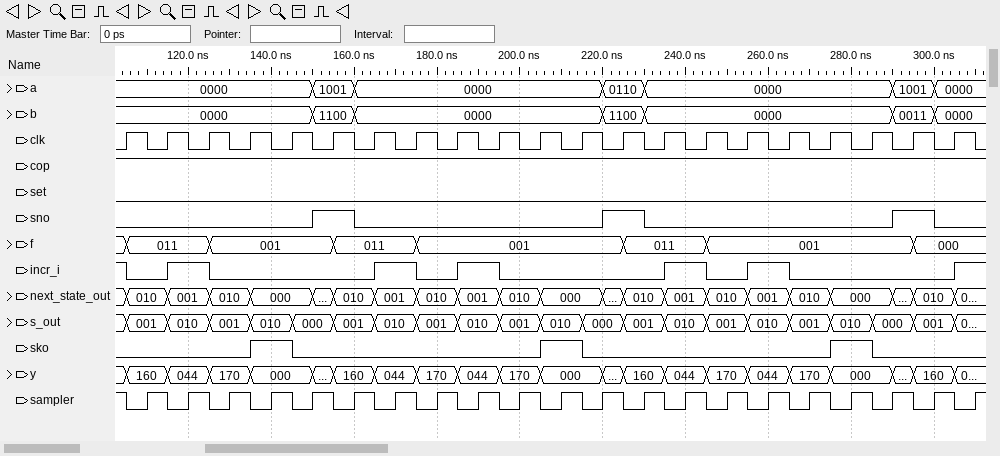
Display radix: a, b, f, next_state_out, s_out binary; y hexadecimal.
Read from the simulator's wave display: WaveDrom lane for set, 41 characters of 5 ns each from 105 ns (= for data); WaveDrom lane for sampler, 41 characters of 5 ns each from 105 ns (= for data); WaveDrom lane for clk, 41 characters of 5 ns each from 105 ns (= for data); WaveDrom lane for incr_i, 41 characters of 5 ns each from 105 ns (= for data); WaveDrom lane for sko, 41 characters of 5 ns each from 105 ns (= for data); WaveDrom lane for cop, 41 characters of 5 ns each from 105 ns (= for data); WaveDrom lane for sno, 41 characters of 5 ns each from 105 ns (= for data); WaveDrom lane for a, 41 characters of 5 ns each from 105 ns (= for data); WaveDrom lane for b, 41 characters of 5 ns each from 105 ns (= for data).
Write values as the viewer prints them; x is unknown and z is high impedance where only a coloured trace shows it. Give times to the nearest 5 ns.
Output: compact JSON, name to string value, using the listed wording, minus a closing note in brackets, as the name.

{"WaveDrom lane for set, 41 characters of 5 ns each from 105 ns": "{name: 'set', wave: '0........................................'}", "WaveDrom lane for sampler, 41 characters of 5 ns each from 105 ns": "{name: 'sampler', wave: '01010101010101010101010101010101010101010'}", "WaveDrom lane for clk, 41 characters of 5 ns each from 105 ns": "{name: 'clk', wave: '10101010101010101010101010101010101010101'}", "WaveDrom lane for incr_i, 41 characters of 5 ns each from 105 ns": "{name: 'incr_i', wave: '0.1.0.......1.0.1.0.......1.0.1.0.......1'}", "WaveDrom lane for sko, 41 characters of 5 ns each from 105 ns": "{name: 'sko', wave: '0.....1.0...........1.0...........1.0....'}", "WaveDrom lane for cop, 41 characters of 5 ns each from 105 ns": "{name: 'cop', wave: '1........................................'}", "WaveDrom lane for sno, 41 characters of 5 ns each from 105 ns": "{name: 'sno', wave: '0........1.0...........1.0...........1.0.'}", "WaveDrom lane for a, 41 characters of 5 ns each from 105 ns": "{name: 'a', wave: '=........=.=...........=.=...........=.=.', data: '0000 1001 0000 0110 0000 1001 0000'}", "WaveDrom lane for b, 41 characters of 5 ns each from 105 ns": "{name: 'b', wave: '=........=.=...........=.=...........=.=.', data: '0000 1100 0000 1100 0000 0011 0000'}"}
